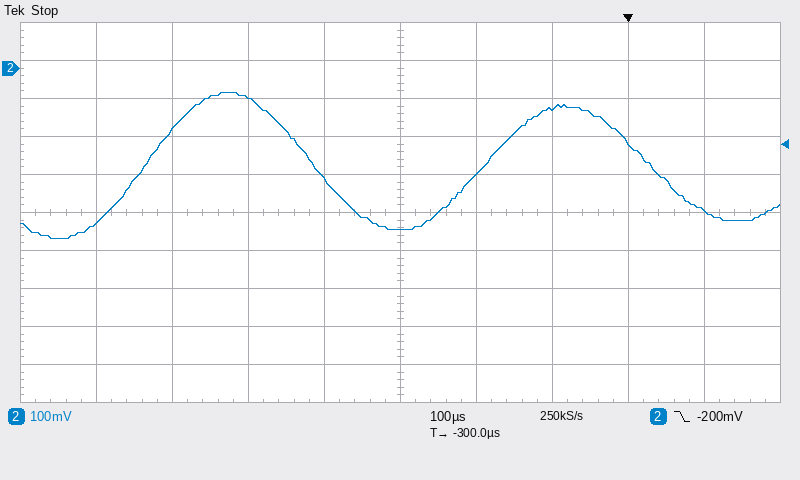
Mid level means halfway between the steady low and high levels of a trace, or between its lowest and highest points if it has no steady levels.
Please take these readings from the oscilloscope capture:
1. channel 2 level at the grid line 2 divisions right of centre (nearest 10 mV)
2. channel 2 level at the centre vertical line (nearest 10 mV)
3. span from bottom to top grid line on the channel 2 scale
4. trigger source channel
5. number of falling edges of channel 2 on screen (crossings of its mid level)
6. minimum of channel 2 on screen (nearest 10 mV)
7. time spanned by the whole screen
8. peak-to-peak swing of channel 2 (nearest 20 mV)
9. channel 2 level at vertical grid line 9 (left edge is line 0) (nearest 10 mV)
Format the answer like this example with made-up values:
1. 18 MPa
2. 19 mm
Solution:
1. -110 mV
2. -420 mV
3. 1 V
4. channel 2
5. 2
6. -450 mV
7. 1 ms
8. 380 mV
9. -380 mV
